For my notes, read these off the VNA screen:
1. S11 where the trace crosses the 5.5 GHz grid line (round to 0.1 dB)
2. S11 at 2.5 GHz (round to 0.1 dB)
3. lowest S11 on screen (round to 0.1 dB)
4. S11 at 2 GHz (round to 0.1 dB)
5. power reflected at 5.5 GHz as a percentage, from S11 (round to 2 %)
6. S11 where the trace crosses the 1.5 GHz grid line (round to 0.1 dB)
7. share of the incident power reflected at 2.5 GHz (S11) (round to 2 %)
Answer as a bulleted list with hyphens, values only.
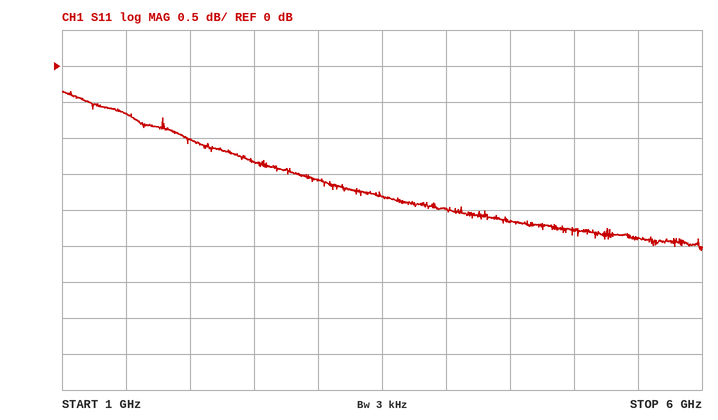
- -2.4 dB
- -1.3 dB
- -2.6 dB
- -1.0 dB
- 58 %
- -0.7 dB
- 74 %
